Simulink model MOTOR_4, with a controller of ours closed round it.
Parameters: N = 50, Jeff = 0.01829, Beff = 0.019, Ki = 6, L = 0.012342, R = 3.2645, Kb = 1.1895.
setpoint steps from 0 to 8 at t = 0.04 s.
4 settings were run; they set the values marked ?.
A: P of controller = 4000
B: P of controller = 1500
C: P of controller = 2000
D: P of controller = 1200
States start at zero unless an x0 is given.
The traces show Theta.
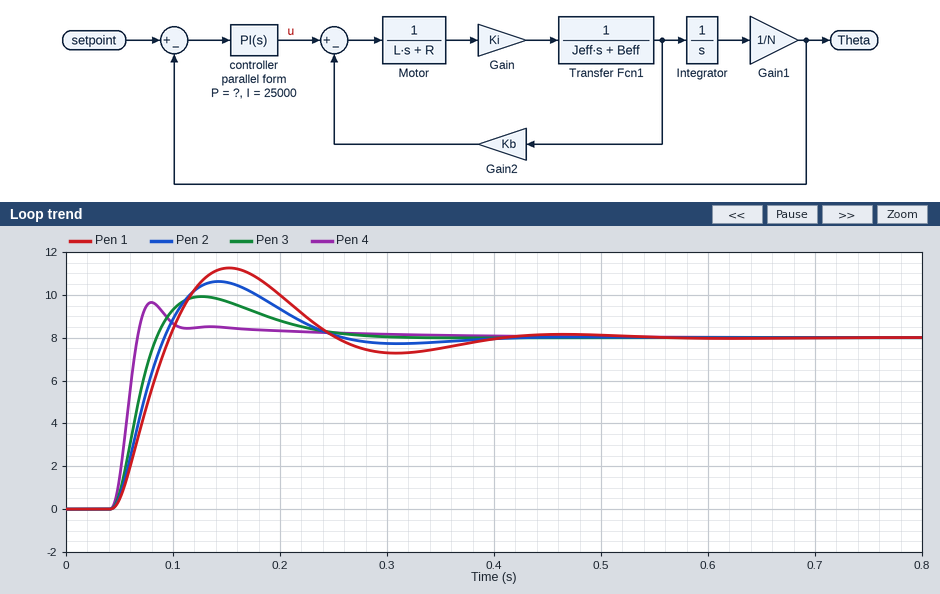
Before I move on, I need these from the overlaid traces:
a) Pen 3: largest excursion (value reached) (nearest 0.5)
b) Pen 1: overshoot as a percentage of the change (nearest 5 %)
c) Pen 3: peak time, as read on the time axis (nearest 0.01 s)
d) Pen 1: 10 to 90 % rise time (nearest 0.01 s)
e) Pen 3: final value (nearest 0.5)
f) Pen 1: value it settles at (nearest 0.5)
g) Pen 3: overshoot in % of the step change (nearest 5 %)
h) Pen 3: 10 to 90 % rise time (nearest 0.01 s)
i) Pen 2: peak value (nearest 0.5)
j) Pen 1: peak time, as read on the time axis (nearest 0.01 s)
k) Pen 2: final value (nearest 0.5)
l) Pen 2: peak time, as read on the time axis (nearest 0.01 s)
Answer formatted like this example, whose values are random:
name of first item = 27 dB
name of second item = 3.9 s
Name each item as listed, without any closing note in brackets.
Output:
Pen 3: largest excursion (value reached) = 10.0
Pen 1: overshoot as a percentage of the change = 40 %
Pen 3: peak time, as read on the time axis = 0.13 s
Pen 1: 10 to 90 % rise time = 0.04 s
Pen 3: final value = 8.0
Pen 1: value it settles at = 8.0
Pen 3: overshoot in % of the step change = 25 %
Pen 3: 10 to 90 % rise time = 0.03 s
Pen 2: peak value = 10.5
Pen 1: peak time, as read on the time axis = 0.15 s
Pen 2: final value = 8.0
Pen 2: peak time, as read on the time axis = 0.14 s
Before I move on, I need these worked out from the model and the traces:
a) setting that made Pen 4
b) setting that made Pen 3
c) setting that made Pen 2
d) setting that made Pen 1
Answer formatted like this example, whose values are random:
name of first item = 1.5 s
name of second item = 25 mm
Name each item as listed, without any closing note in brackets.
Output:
setting that made Pen 4 = A
setting that made Pen 3 = C
setting that made Pen 2 = B
setting that made Pen 1 = D
